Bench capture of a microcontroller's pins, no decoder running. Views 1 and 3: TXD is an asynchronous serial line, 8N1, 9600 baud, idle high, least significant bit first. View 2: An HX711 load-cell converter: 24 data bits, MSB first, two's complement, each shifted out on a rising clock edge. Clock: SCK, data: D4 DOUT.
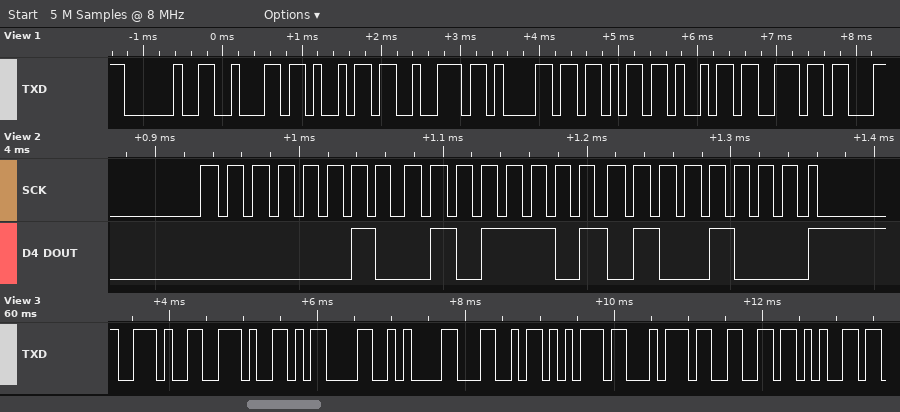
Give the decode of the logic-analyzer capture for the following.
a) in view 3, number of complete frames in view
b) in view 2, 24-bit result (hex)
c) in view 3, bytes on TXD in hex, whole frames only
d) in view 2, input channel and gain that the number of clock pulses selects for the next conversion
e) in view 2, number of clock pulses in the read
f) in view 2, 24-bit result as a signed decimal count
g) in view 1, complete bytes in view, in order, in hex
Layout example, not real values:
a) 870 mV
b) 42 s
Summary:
a) 9
b) 0x025D48
c) 2E 2E 0D 0A 4C 75 74 66 65
d) channel A, gain 128
e) 25
f) 154952
g) 20 62 69 72 61 6B 69 6E
